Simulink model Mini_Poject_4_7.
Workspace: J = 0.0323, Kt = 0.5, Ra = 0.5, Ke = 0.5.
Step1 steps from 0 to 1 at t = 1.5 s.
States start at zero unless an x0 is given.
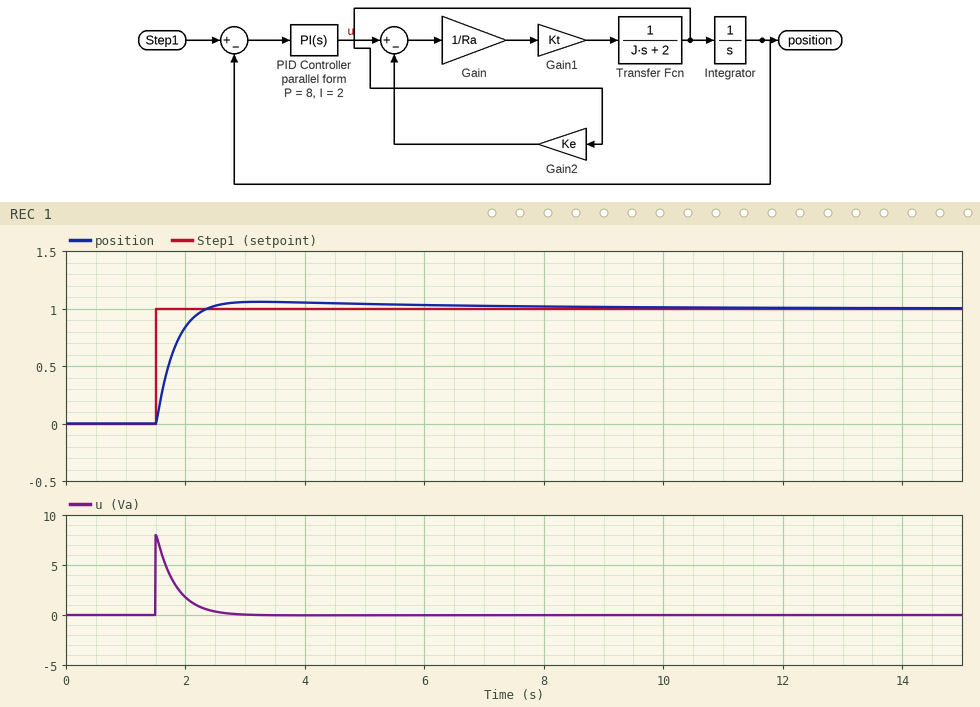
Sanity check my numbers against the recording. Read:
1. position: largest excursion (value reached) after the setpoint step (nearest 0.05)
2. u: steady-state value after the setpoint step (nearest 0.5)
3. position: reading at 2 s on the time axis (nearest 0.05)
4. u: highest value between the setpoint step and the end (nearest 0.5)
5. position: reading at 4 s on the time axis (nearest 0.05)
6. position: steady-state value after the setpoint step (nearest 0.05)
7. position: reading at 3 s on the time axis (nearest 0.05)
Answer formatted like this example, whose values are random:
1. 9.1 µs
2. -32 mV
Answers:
1. 1.05
2. 0.0
3. 0.85
4. 8.0
5. 1.05
6. 1.00
7. 1.05
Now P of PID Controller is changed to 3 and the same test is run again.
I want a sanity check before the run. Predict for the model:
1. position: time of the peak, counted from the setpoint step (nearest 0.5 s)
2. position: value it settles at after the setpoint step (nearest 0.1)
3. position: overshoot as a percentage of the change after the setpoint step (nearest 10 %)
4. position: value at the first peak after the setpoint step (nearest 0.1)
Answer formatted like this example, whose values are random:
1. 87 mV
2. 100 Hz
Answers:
1. 2.5 s
2. 1.0
3. 20 %
4. 1.2
